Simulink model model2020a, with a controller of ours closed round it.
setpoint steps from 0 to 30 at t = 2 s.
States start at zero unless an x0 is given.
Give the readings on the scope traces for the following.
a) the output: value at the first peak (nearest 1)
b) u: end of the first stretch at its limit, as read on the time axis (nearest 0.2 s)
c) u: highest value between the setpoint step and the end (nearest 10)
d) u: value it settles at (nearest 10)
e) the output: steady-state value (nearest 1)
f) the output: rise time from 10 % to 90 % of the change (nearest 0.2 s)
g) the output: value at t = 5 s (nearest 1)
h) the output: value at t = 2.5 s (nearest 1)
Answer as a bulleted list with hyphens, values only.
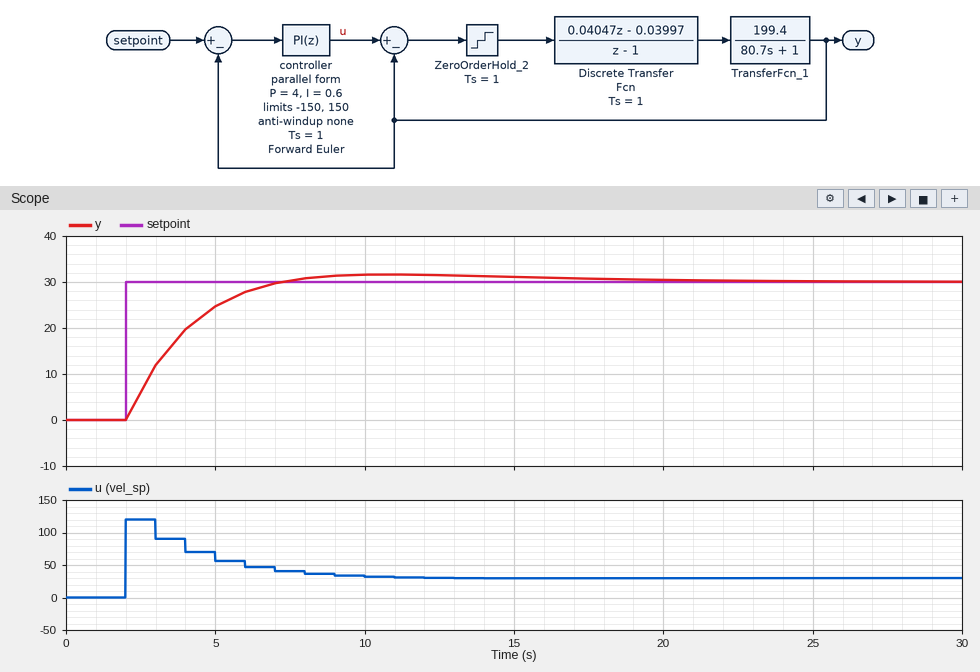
- 32
- 3.0 s
- 120
- 30
- 30
- 3.4 s
- 25
- 6
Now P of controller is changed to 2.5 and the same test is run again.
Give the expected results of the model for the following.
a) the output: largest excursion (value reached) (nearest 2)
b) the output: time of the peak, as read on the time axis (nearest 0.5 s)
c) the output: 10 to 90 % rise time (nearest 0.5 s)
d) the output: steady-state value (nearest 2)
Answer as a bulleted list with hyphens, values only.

- 34
- 12.0 s
- 4.5 s
- 30
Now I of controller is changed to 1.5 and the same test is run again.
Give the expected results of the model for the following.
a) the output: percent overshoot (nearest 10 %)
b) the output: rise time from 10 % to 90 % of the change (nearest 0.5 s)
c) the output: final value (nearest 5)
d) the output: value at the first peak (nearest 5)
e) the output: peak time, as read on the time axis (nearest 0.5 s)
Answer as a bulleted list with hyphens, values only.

- 30 %
- 2.5 s
- 30
- 40
- 8.0 s
